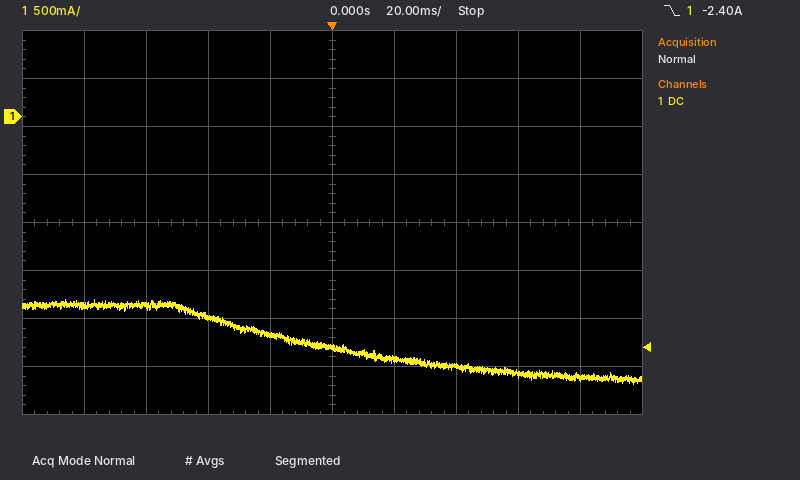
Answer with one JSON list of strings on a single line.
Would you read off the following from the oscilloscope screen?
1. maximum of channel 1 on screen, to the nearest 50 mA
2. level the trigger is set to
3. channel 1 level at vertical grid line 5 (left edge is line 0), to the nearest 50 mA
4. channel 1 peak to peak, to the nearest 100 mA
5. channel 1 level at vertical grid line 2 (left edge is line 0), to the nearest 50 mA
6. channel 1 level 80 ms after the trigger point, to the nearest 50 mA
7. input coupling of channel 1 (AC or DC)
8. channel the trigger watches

["-1.90 A", "-2.40 A", "-2.40 A", "900 mA", "-1.95 A", "-2.70 A", "DC", "channel 1"]
